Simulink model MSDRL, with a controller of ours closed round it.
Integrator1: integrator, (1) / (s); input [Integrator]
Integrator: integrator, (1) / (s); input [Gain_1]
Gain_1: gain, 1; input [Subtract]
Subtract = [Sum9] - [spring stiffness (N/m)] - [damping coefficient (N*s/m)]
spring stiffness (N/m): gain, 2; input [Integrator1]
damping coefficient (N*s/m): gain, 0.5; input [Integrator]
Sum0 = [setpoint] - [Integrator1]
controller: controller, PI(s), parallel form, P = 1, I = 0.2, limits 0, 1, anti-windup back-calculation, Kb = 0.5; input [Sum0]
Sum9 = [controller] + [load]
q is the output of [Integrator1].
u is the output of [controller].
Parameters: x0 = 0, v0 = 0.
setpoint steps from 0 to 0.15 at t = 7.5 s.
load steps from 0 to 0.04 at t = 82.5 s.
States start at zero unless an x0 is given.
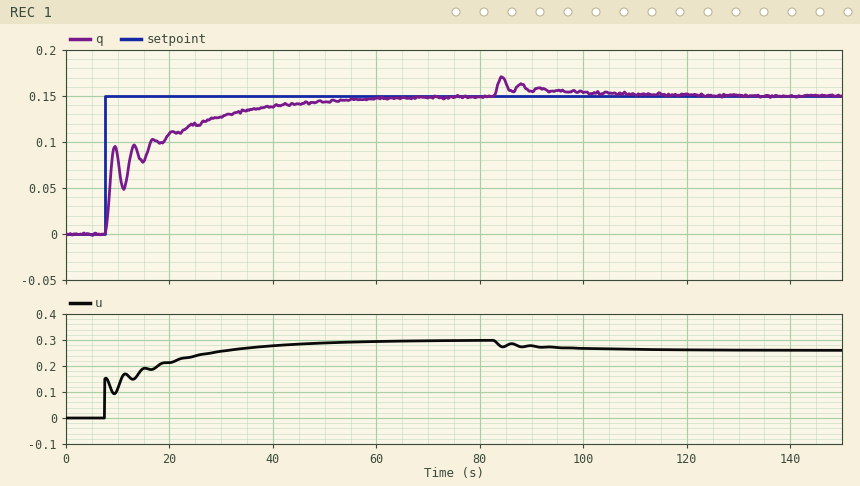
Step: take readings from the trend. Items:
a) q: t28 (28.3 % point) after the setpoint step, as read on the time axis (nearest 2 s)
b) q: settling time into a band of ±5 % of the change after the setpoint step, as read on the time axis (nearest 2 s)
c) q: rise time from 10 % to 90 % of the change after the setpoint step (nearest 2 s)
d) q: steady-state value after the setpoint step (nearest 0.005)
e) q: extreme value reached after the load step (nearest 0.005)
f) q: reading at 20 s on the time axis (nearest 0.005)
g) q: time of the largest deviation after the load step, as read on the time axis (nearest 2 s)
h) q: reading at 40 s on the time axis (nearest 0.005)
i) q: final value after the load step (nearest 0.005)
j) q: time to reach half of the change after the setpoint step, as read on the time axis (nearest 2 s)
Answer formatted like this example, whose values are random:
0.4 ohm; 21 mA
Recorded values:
8 s; 46 s; 28 s; 0.150; 0.170; 0.110; 84 s; 0.140; 0.150; 8 s
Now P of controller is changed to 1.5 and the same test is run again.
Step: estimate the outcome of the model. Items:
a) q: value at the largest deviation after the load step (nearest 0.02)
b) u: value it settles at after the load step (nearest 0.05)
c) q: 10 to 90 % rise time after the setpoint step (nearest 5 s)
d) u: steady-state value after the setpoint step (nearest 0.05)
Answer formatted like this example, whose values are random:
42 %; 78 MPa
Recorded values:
0.16; 0.25; 30 s; 0.30
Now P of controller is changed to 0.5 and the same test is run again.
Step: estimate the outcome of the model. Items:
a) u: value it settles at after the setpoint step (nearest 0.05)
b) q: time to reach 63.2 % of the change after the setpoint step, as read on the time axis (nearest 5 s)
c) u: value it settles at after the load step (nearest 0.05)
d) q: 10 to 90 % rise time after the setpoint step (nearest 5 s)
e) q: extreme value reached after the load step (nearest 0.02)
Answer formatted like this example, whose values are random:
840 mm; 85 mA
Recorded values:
0.30; 15 s; 0.25; 25 s; 0.18
